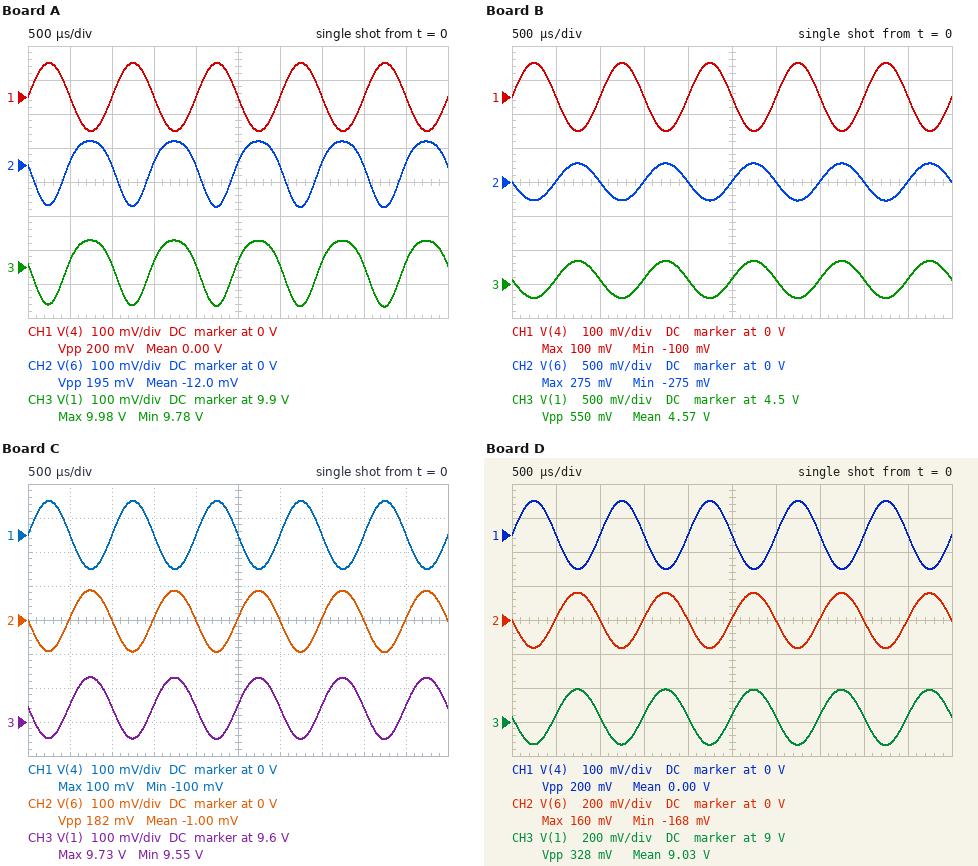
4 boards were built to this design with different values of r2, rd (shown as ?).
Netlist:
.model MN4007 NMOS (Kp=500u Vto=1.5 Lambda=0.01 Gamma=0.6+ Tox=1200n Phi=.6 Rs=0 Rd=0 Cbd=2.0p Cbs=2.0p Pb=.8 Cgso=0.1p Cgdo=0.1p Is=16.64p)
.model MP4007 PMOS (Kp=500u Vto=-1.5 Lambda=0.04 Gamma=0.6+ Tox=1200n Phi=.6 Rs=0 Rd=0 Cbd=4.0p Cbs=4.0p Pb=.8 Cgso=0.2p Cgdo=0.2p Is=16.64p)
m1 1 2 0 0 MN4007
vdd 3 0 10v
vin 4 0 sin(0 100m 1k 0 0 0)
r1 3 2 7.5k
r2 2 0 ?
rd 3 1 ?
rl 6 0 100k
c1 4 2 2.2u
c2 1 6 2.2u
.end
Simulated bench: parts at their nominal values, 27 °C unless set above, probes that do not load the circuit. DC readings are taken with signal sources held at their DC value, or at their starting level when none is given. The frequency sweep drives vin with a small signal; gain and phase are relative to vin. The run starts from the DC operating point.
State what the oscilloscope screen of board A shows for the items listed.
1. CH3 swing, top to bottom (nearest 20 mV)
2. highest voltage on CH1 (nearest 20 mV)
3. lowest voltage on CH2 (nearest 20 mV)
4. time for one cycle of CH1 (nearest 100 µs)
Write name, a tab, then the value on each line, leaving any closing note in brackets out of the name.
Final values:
CH3 swing, top to bottom	200 mV
highest voltage on CH1	100 mV
lowest voltage on CH2	-120 mV
time for one cycle of CH1	1.0 ms
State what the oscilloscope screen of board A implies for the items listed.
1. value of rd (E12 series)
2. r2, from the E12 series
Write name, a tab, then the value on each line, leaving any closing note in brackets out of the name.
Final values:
value of rd	12 kΩ
r2, from the E12 series	1.5 kΩ
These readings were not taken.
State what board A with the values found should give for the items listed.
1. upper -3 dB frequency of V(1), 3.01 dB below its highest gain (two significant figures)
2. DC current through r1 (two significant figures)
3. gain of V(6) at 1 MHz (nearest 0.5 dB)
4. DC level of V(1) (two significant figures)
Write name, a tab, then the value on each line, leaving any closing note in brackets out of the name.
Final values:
upper -3 dB frequency of V(1), 3.01 dB below its highest gain	27 MHz
DC current through r1	1.1 mA
gain of V(6) at 1 MHz	0 dB
DC level of V(1)	9.9 V
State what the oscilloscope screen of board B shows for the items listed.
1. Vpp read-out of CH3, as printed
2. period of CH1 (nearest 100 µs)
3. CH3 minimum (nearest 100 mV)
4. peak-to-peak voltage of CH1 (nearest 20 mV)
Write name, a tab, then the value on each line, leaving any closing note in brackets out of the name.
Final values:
Vpp read-out of CH3, as printed	550 mV
period of CH1	1.0 ms
CH3 minimum	4.3 V
peak-to-peak voltage of CH1	200 mV
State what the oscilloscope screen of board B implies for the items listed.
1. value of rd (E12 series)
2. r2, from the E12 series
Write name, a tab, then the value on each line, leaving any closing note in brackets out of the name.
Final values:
value of rd	1.5 kΩ
r2, from the E12 series	8.2 kΩ
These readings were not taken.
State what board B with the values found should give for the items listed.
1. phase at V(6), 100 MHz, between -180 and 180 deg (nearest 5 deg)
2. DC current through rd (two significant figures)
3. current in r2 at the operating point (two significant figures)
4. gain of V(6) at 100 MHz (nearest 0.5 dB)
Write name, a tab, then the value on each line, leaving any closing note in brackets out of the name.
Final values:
phase at V(6), 100 MHz, between -180 and 180 deg	145 deg
DC current through rd	3.6 mA
current in r2 at the operating point	640 µA
gain of V(6) at 100 MHz	7.0 dB
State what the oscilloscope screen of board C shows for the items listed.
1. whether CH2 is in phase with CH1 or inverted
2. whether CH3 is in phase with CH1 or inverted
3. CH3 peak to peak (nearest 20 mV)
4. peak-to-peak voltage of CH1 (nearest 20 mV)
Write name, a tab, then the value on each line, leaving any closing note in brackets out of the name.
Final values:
whether CH2 is in phase with CH1 or inverted	inverted
whether CH3 is in phase with CH1 or inverted	inverted
CH3 peak to peak	180 mV
peak-to-peak voltage of CH1	200 mV
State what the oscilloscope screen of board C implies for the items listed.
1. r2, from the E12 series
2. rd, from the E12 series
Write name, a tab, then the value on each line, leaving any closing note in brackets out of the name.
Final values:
r2, from the E12 series	2.2 kΩ
rd, from the E12 series	2.2 kΩ
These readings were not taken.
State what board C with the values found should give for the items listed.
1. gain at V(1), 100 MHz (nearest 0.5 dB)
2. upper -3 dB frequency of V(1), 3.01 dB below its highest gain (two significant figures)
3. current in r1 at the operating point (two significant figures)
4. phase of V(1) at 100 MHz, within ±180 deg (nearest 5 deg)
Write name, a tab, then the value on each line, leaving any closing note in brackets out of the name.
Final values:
gain at V(1), 100 MHz	-3.0 dB
upper -3 dB frequency of V(1), 3.01 dB below its highest gain	130 MHz
current in r1 at the operating point	1.0 mA
phase of V(1) at 100 MHz, within ±180 deg	145 deg
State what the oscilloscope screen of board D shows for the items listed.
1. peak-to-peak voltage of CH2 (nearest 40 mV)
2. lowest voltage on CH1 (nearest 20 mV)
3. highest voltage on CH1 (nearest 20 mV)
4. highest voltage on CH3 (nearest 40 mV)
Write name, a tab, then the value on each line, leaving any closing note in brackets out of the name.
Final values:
peak-to-peak voltage of CH2	320 mV
lowest voltage on CH1	-100 mV
highest voltage on CH1	100 mV
highest voltage on CH3	9.20 V
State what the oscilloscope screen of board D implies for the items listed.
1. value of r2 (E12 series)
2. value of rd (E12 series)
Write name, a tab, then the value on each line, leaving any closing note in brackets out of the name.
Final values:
value of r2	2.7 kΩ
value of rd	2.7 kΩ
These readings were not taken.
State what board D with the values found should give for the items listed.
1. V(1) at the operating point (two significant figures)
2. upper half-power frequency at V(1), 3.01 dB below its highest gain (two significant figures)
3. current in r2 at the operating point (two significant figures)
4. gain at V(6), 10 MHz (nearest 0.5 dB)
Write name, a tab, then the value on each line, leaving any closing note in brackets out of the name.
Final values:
V(1) at the operating point	9.0 V
upper half-power frequency at V(1), 3.01 dB below its highest gain	110 MHz
current in r2 at the operating point	980 µA
gain at V(6), 10 MHz	4.0 dB
